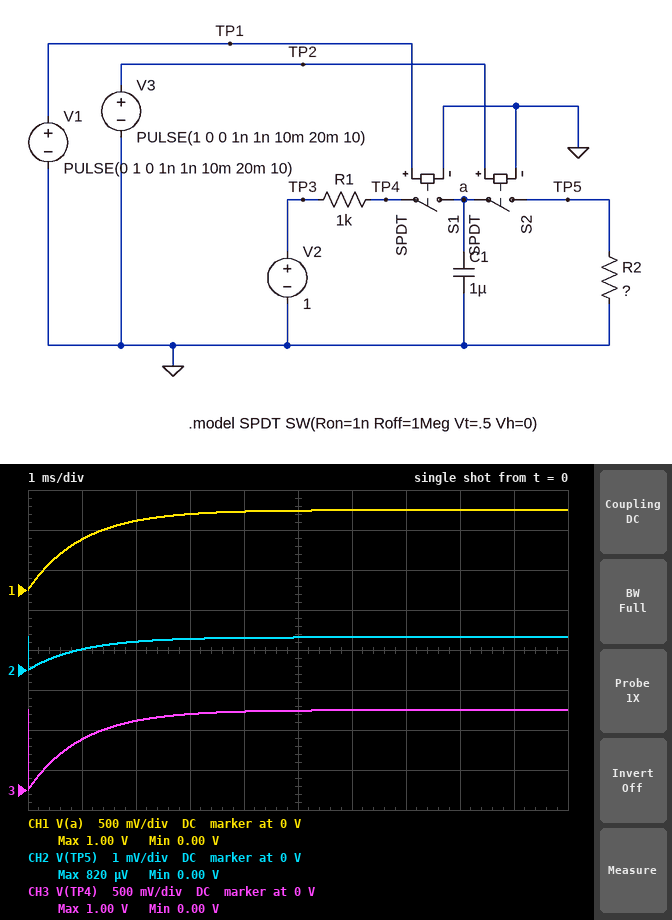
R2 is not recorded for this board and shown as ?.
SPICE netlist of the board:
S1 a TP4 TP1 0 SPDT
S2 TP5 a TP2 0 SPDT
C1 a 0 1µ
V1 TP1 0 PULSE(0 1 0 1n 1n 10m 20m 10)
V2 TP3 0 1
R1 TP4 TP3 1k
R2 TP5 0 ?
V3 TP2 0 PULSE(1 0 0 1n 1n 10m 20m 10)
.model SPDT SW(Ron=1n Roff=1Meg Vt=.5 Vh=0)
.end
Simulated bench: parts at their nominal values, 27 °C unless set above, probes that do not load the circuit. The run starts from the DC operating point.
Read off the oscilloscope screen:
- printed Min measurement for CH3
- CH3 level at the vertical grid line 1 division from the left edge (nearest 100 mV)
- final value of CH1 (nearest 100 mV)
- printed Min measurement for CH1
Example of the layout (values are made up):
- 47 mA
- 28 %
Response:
- 0.00 V
- 600 mV
- 1.0 V
- 0.00 V
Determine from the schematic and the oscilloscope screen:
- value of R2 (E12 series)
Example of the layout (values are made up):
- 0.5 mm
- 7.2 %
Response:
- 820 Ω
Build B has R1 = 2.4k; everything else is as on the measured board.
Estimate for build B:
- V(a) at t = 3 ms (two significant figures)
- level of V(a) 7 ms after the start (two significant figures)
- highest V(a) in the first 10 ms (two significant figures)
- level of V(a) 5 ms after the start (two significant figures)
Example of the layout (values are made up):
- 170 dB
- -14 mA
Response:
- 710 mV
- 940 mV
- 980 mV
- 870 mV
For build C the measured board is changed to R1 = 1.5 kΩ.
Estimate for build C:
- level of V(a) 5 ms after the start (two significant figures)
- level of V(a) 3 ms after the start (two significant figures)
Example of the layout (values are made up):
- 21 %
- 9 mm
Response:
- 960 mV
- 860 mV
